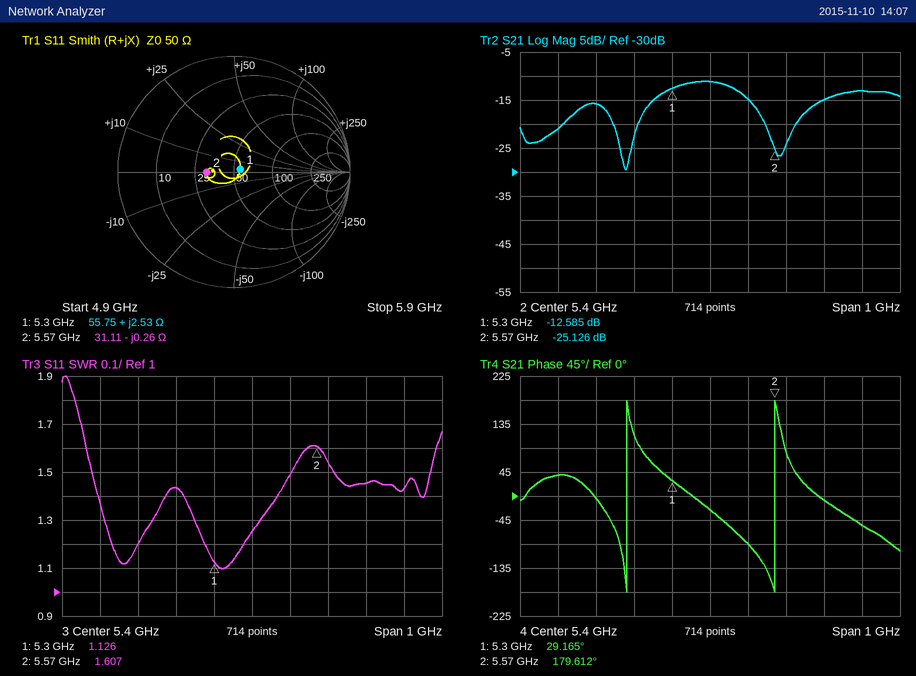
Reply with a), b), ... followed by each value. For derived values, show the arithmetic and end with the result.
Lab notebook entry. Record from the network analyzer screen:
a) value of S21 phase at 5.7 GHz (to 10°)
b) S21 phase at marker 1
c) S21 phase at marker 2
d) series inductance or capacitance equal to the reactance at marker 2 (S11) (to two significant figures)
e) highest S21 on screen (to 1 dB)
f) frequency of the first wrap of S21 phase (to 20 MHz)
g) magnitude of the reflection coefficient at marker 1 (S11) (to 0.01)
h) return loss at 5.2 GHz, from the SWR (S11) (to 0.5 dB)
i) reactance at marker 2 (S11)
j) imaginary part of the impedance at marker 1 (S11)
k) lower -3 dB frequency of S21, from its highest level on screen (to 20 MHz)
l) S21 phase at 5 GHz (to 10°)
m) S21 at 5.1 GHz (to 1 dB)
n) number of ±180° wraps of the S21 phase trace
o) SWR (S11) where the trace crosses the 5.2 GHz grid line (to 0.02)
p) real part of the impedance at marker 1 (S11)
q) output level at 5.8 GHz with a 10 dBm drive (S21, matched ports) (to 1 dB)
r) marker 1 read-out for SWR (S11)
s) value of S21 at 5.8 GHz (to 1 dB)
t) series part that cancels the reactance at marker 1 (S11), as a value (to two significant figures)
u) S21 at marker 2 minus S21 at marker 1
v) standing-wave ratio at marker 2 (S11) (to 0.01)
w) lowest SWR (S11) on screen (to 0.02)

a) -10°
b) 29.165°
c) 179.612°
d) C = 1/(2π × 5.57 GHz × 0.26 Ω) ≈ 110 pF
e) -11 dB
f) 5.18 GHz
g) 0.06
h) −20 log10((1.44 − 1)/(1.44 + 1)) ≈ 14.9 dB, so 15.0 dB to the nearest 0.5 dB
i) -0.26 Ω
j) +2.53 Ω
k) 5.26 GHz
l) 40°
m) -16 dB
n) 2
o) 1.44
p) 55.75 Ω
q) 10 dBm + (-13 dB) = -3 dBm
r) 1.126
s) -13 dB
t) C = 1/(2π × 5.3 GHz × 2.53 Ω) ≈ 12 pF
u) -25.126 − (-12.585) = -12.541 dB
v) 1.61
w) 1.10
